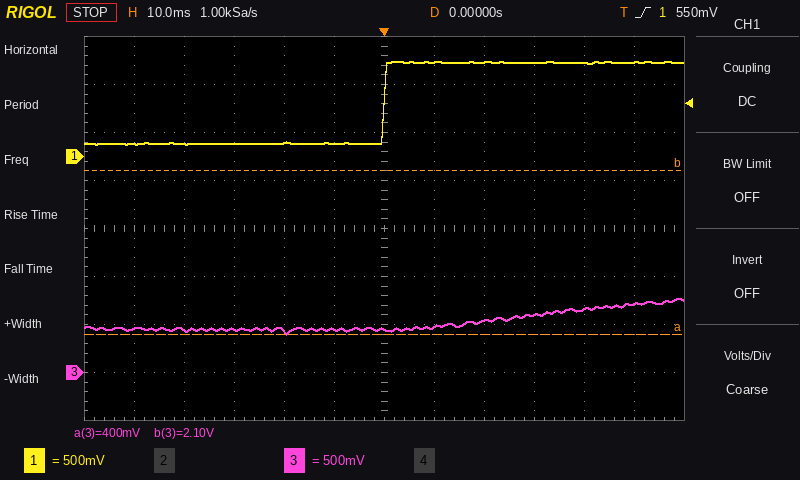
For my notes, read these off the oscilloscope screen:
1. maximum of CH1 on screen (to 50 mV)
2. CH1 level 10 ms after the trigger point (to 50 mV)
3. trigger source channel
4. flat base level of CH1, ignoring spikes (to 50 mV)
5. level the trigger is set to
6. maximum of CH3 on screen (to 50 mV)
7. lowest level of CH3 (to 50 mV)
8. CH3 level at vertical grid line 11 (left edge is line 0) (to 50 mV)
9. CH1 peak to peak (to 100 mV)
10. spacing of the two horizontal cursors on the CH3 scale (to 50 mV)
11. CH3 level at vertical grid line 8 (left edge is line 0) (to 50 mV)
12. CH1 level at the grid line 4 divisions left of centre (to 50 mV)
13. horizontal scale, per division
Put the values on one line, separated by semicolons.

1.00 V; 1.00 V; CH1; 150 mV; 550 mV; 750 mV; 400 mV; 700 mV; 900 mV; 1.70 V; 550 mV; 150 mV; 10 ms
